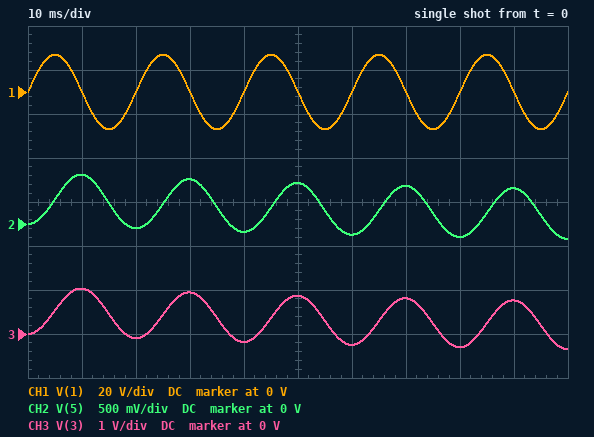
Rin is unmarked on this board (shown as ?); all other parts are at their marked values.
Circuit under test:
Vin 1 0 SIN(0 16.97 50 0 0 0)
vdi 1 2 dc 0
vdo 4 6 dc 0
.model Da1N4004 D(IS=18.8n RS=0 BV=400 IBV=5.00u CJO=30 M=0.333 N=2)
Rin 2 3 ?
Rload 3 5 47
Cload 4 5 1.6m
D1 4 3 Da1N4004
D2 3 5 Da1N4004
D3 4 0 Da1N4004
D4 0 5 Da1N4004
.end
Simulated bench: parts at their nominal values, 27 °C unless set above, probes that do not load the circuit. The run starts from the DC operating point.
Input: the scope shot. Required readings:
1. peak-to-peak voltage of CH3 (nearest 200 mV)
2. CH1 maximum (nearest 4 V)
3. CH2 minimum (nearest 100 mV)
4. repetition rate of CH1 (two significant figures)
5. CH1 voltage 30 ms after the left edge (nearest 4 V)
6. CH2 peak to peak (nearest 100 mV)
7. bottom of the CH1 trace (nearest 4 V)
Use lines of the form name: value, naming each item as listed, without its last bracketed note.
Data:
peak-to-peak voltage of CH3: 1.4 V
CH1 maximum: 16 V
CH2 minimum: -200 mV
repetition rate of CH1: 50 Hz
CH1 voltage 30 ms after the left edge: 0 V
CH2 peak to peak: 700 mV
bottom of the CH1 trace: -16 V
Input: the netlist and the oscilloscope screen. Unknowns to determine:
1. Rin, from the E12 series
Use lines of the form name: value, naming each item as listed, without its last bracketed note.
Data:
Rin, from the E12 series: 3.3 mΩ
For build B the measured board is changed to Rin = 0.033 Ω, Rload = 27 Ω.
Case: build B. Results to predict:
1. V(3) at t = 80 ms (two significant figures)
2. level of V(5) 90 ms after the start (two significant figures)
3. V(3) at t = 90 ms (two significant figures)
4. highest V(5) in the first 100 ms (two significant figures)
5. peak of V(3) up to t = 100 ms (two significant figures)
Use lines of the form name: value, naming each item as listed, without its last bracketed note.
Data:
V(3) at t = 80 ms: -4.2 mV
level of V(5) 90 ms after the start: 53 mV
V(3) at t = 90 ms: 100 mV
highest V(5) in the first 100 ms: 55 mV
peak of V(3) up to t = 100 ms: 110 mV
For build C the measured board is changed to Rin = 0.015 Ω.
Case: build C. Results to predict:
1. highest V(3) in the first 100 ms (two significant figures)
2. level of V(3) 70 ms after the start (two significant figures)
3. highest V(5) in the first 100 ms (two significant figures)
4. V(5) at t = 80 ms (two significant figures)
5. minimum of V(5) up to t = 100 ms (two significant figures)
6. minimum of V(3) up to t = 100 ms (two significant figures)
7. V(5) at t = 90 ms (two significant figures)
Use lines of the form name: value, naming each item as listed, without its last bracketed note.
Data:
highest V(3) in the first 100 ms: 240 mV
level of V(3) 70 ms after the start: 220 mV
highest V(5) in the first 100 ms: 120 mV
V(5) at t = 80 ms: -9.8 mV
minimum of V(5) up to t = 100 ms: -12 mV
minimum of V(3) up to t = 100 ms: -24 mV
V(5) at t = 90 ms: 110 mV
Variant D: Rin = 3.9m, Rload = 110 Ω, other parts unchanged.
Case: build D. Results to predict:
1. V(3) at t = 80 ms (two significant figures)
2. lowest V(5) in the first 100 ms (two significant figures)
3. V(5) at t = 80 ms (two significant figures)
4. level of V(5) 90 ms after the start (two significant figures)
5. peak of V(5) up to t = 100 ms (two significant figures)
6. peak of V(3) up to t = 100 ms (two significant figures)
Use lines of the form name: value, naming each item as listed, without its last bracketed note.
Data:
V(3) at t = 80 ms: -230 mV
lowest V(5) in the first 100 ms: -130 mV
V(5) at t = 80 ms: -110 mV
level of V(5) 90 ms after the start: 360 mV
peak of V(5) up to t = 100 ms: 470 mV
peak of V(3) up to t = 100 ms: 880 mV
